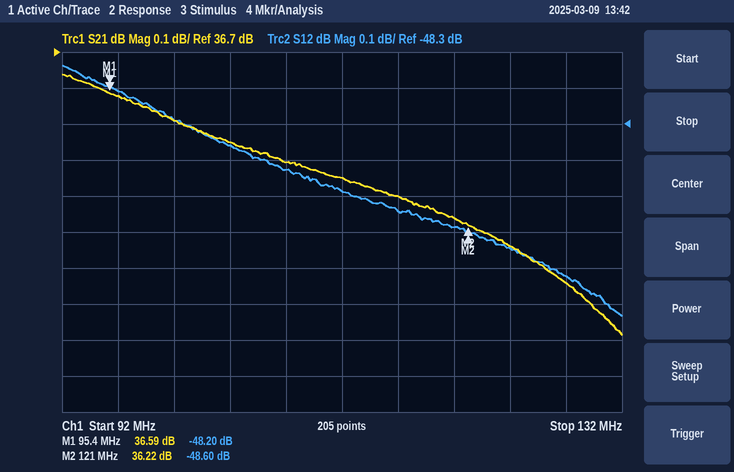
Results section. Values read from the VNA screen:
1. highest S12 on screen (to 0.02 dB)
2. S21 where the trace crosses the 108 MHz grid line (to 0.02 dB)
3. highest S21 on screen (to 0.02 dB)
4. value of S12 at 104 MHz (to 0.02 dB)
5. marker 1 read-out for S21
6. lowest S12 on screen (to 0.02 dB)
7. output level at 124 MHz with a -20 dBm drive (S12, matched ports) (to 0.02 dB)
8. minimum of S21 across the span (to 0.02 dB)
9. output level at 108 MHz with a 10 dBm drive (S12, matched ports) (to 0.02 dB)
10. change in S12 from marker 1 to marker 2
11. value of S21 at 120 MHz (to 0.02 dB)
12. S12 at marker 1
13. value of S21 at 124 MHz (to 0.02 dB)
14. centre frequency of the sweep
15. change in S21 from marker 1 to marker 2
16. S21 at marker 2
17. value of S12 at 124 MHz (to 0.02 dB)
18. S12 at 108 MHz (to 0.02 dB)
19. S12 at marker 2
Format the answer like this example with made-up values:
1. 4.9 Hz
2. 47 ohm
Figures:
1. -48.14 dB
2. 36.40 dB
3. 36.64 dB
4. -48.36 dB
5. 36.59 dB
6. -48.84 dB
7. -68.64 dBm
8. 35.92 dB
9. -38.42 dBm
10. -0.40 dB
11. 36.24 dB
12. -48.20 dB
13. 36.16 dB
14. 112 MHz
15. -0.37 dB
16. 36.22 dB
17. -48.64 dB
18. -48.42 dB
19. -48.60 dB
